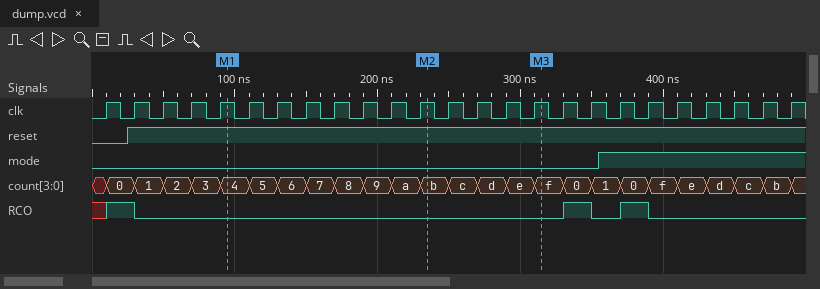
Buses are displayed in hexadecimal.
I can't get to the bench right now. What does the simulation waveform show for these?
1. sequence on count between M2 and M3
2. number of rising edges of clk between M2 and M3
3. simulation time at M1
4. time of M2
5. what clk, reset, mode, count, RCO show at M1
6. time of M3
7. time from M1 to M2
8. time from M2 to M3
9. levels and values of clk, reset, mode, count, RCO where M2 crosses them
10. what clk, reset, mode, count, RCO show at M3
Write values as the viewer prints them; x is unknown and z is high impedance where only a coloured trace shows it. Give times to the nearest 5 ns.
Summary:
b, c, d, e, f
4
95 ns
235 ns
clk=1, reset=1, mode=0, count=4, RCO=0
315 ns
140 ns
80 ns
clk=1, reset=1, mode=0, count=b, RCO=0
clk=1, reset=1, mode=0, count=f, RCO=0
